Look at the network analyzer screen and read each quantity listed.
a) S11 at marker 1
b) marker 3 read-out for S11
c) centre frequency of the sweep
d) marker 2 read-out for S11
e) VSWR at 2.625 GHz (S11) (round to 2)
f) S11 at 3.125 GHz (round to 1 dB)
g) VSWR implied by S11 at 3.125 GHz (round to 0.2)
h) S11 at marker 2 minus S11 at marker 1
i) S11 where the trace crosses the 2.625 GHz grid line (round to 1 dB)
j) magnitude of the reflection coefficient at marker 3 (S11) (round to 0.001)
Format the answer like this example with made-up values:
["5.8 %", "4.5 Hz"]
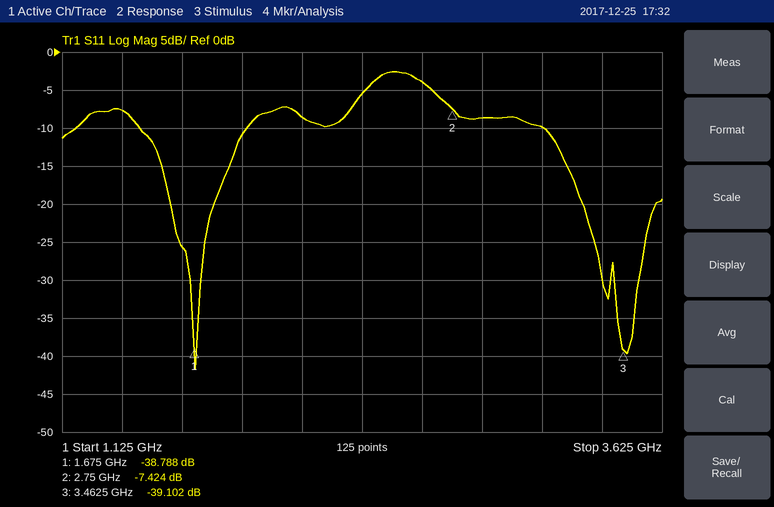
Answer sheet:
["-38.788 dB", "-39.102 dB", "2.375 GHz", "-7.424 dB", "4", "-10 dB", "2.0", "31.364 dB", "-4 dB", "0.011"]
